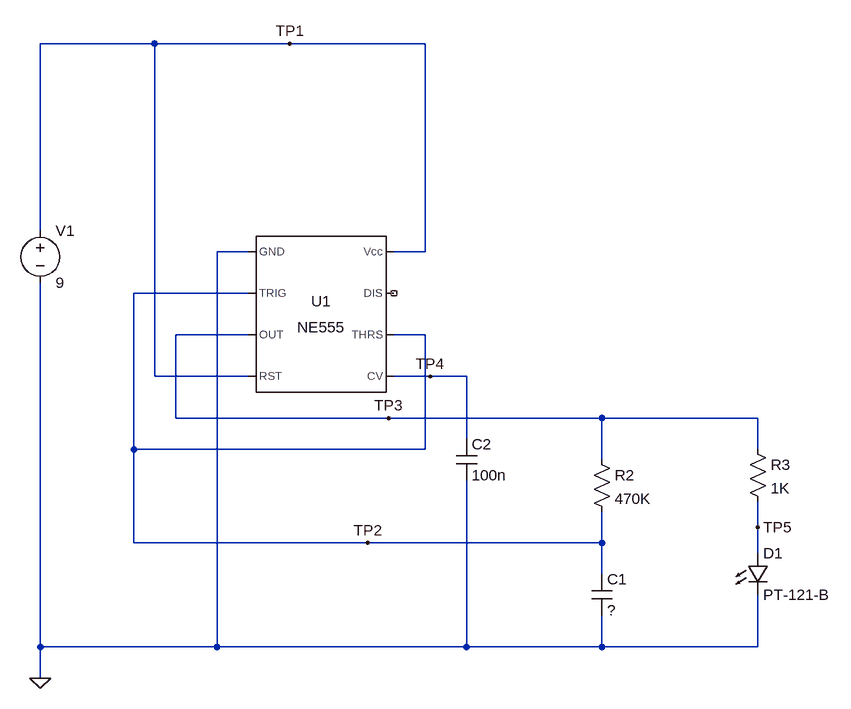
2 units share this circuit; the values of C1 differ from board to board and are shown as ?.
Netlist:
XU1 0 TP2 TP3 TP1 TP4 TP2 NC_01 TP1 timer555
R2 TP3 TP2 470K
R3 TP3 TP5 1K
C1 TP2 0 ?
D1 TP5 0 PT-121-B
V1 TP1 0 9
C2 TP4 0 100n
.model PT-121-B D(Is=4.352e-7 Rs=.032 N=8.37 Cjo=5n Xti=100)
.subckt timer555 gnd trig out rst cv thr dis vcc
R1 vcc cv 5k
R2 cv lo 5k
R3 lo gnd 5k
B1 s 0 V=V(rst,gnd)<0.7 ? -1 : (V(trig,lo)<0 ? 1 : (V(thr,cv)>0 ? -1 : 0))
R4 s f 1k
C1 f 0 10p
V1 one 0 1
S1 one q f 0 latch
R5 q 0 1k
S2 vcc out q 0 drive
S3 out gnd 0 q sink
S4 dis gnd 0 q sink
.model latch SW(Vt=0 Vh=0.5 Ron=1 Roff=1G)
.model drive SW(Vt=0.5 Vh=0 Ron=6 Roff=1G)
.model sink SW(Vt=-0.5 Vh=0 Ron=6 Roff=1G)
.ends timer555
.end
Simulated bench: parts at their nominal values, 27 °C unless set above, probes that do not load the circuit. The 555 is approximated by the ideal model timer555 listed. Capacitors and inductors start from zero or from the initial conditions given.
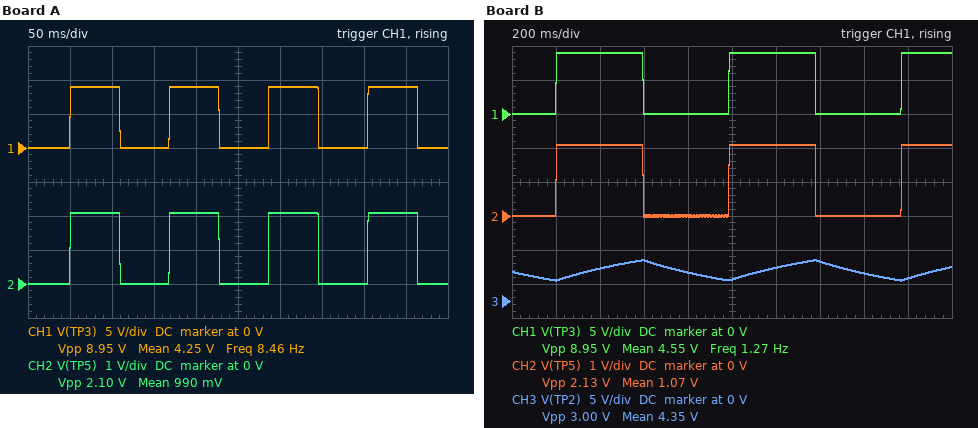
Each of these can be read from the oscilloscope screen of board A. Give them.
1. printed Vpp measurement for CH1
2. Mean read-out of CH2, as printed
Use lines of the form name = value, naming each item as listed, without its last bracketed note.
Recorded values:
printed Vpp measurement for CH1 = 8.95 V
Mean read-out of CH2, as printed = 990 mV
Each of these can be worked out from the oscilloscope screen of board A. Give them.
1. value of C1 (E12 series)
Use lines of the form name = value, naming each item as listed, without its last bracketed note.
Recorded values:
value of C1 = 180 nF
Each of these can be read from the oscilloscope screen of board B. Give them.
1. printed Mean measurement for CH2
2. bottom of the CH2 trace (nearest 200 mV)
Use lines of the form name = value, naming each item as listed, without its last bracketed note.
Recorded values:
printed Mean measurement for CH2 = 1.07 V
bottom of the CH2 trace = 0 V
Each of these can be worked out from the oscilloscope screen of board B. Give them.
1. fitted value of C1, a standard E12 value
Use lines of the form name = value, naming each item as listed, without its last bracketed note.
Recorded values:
fitted value of C1, a standard E12 value = 1.2 µF
